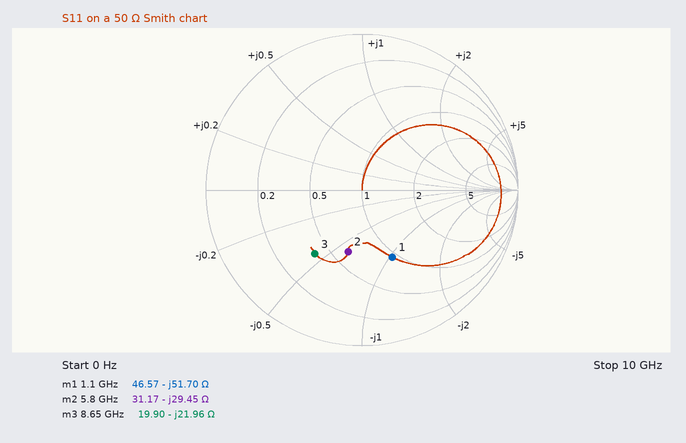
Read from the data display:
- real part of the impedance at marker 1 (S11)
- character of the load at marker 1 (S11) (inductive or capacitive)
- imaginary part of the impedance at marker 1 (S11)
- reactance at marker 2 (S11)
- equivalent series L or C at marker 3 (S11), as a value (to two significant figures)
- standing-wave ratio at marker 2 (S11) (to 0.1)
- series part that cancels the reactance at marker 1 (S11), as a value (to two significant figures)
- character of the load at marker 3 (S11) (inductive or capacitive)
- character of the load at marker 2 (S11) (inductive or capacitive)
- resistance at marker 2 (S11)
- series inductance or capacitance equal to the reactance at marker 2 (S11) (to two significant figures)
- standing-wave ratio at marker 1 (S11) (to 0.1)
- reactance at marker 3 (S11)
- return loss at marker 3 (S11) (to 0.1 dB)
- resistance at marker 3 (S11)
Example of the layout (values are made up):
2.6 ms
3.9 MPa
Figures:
46.57 Ω
capacitive
-51.70 Ω
-29.45 Ω
840 fF
2.4
7.5 nH
capacitive
capacitive
31.17 Ω
930 fF
2.8
-21.96 Ω
5.9 dB
19.90 Ω
